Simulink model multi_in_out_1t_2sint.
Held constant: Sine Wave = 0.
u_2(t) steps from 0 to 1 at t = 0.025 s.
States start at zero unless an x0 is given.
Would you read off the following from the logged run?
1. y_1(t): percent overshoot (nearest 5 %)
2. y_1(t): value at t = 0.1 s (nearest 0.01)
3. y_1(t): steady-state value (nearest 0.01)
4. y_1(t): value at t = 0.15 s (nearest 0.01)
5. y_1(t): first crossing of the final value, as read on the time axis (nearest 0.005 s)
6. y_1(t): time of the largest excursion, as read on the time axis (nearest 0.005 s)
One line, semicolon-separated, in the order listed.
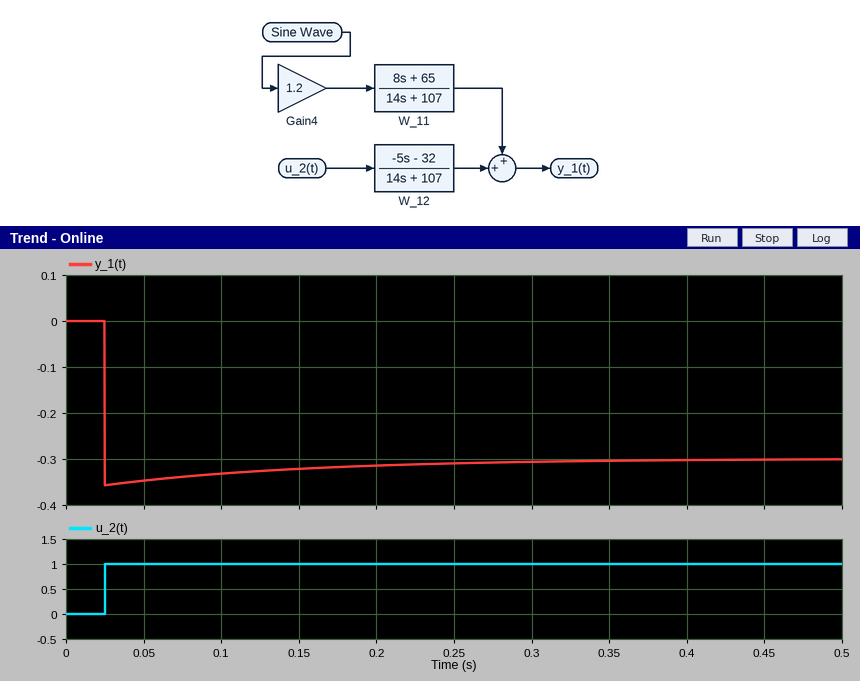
20 %; -0.33; -0.30; -0.32; 0.025 s; 0.025 s
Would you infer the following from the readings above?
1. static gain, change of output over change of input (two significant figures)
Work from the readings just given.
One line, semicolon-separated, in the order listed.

-0.30
